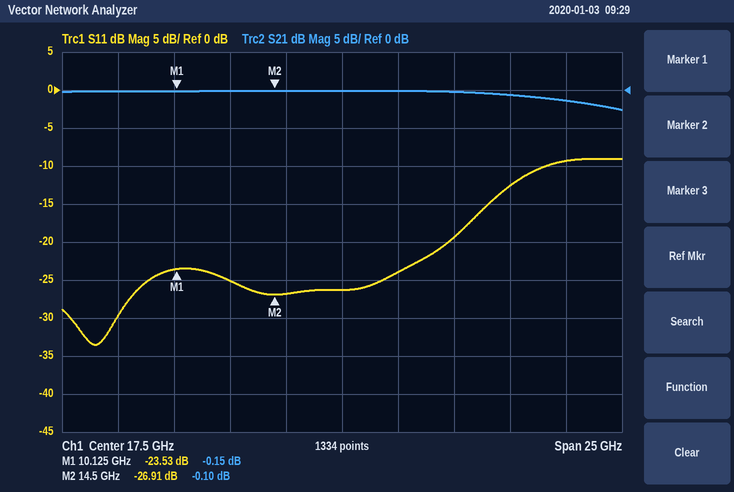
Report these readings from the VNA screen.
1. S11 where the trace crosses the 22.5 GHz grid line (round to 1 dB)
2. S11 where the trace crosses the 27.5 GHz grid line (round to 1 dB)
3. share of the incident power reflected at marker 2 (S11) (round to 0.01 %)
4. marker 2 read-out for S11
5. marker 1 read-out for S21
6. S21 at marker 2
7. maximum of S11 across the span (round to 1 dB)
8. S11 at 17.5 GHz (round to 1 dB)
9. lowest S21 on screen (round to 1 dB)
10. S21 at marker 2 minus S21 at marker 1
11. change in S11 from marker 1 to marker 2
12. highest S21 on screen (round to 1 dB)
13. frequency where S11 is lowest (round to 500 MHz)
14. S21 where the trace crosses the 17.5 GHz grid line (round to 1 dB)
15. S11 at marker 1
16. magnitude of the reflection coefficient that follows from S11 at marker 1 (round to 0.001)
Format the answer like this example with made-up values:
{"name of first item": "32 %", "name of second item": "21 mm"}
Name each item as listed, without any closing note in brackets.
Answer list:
{"S11 where the trace crosses the 22.5 GHz grid line": "-19 dB", "S11 where the trace crosses the 27.5 GHz grid line": "-9 dB", "share of the incident power reflected at marker 2 (S11)": "0.20 %", "marker 2 read-out for S11": "-26.91 dB", "marker 1 read-out for S21": "-0.15 dB", "S21 at marker 2": "-0.10 dB", "maximum of S11 across the span": "-9 dB", "S11 at 17.5 GHz": "-26 dB", "lowest S21 on screen": "-3 dB", "S21 at marker 2 minus S21 at marker 1": "0.05 dB", "change in S11 from marker 1 to marker 2": "-3.38 dB", "highest S21 on screen": "0 dB", "frequency where S11 is lowest": "6.5 GHz", "S21 where the trace crosses the 17.5 GHz grid line": "0 dB", "S11 at marker 1": "-23.53 dB", "magnitude of the reflection coefficient that follows from S11 at marker 1": "0.067"}
